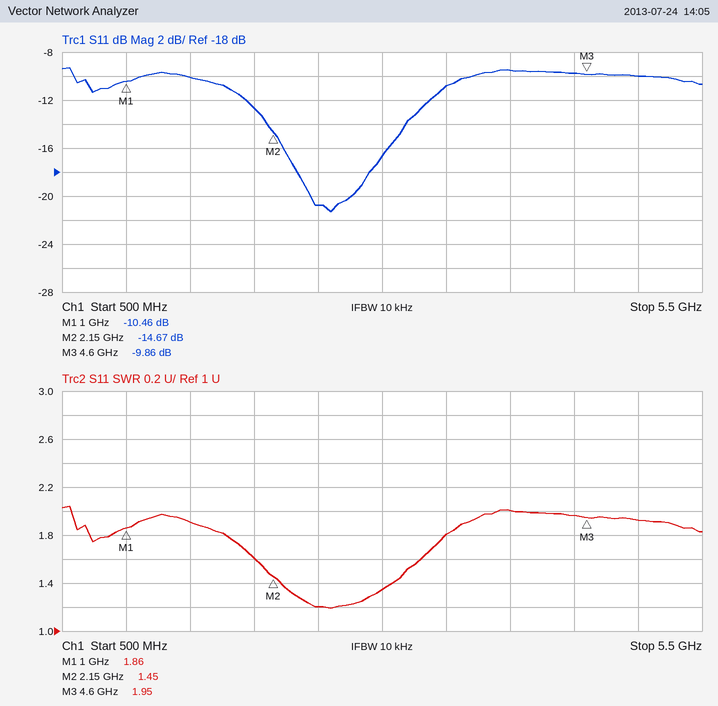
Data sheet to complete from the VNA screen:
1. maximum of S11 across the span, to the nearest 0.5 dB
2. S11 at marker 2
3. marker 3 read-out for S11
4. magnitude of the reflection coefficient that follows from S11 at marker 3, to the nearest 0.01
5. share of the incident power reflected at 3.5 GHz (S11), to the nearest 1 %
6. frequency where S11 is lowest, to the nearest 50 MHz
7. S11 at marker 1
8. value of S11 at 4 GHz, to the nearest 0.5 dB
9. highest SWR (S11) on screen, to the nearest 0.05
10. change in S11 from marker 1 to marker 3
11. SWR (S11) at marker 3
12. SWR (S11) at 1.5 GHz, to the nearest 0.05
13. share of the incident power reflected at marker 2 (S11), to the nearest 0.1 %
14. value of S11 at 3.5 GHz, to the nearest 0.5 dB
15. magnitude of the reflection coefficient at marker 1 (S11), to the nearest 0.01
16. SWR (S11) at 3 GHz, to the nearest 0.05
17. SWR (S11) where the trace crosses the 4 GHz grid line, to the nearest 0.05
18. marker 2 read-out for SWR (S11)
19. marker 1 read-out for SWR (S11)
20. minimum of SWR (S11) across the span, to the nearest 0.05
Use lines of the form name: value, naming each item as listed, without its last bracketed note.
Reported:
maximum of S11 across the span, to the nearest 0.5 dB: -9.5 dB
S11 at marker 2: -14.67 dB
marker 3 read-out for S11: -9.86 dB
magnitude of the reflection coefficient that follows from S11 at marker 3, to the nearest 0.01: 0.32
share of the incident power reflected at 3.5 GHz (S11), to the nearest 1 %: 8 %
frequency where S11 is lowest, to the nearest 50 MHz: 2.60 GHz
S11 at marker 1: -10.46 dB
value of S11 at 4 GHz, to the nearest 0.5 dB: -9.5 dB
highest SWR (S11) on screen, to the nearest 0.05: 2.05
change in S11 from marker 1 to marker 3: 0.60 dB
SWR (S11) at marker 3: 1.95
SWR (S11) at 1.5 GHz, to the nearest 0.05: 1.90
share of the incident power reflected at marker 2 (S11), to the nearest 0.1 %: 3.4 %
value of S11 at 3.5 GHz, to the nearest 0.5 dB: -11.0 dB
magnitude of the reflection coefficient at marker 1 (S11), to the nearest 0.01: 0.30
SWR (S11) at 3 GHz, to the nearest 0.05: 1.35
SWR (S11) where the trace crosses the 4 GHz grid line, to the nearest 0.05: 2.00
marker 2 read-out for SWR: 1.45
marker 1 read-out for SWR: 1.86
minimum of SWR (S11) across the span, to the nearest 0.05: 1.20
